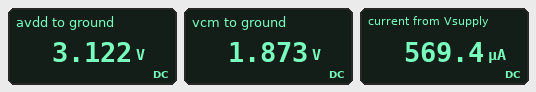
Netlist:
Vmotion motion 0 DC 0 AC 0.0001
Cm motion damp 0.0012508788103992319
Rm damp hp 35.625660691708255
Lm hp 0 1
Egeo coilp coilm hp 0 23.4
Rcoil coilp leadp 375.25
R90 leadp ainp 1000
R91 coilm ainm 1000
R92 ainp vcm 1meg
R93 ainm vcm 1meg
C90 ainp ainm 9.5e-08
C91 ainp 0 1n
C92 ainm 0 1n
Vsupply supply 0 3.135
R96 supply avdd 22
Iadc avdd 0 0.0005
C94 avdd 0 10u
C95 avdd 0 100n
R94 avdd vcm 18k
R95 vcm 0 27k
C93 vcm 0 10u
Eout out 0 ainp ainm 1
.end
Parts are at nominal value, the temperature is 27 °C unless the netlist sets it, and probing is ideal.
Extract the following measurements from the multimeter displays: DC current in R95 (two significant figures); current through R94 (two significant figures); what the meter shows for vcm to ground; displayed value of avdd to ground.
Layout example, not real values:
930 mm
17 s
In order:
69 µA
69 µA
1.873 V
3.122 V
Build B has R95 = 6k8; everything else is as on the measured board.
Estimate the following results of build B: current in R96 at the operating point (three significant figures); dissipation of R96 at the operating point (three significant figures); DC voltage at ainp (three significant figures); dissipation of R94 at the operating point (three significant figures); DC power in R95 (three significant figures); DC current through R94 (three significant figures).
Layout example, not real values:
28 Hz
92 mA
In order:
626 µA
8.62 µW
856 mV
285 µW
108 µW
126 µA
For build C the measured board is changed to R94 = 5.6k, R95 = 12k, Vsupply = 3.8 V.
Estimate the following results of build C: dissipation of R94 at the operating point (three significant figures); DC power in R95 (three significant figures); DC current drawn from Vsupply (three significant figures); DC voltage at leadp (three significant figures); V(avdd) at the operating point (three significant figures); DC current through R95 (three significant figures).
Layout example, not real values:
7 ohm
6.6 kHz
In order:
259 µW
555 µW
715 µA
2.58 V
3.78 V
215 µA
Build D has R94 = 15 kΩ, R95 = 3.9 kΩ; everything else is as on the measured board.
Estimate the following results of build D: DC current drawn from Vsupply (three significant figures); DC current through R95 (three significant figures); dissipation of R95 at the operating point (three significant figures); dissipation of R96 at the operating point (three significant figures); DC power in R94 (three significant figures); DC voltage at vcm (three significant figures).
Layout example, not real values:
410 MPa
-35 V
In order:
665 µA
165 µA
106 µW
9.73 µW
409 µW
644 mV
